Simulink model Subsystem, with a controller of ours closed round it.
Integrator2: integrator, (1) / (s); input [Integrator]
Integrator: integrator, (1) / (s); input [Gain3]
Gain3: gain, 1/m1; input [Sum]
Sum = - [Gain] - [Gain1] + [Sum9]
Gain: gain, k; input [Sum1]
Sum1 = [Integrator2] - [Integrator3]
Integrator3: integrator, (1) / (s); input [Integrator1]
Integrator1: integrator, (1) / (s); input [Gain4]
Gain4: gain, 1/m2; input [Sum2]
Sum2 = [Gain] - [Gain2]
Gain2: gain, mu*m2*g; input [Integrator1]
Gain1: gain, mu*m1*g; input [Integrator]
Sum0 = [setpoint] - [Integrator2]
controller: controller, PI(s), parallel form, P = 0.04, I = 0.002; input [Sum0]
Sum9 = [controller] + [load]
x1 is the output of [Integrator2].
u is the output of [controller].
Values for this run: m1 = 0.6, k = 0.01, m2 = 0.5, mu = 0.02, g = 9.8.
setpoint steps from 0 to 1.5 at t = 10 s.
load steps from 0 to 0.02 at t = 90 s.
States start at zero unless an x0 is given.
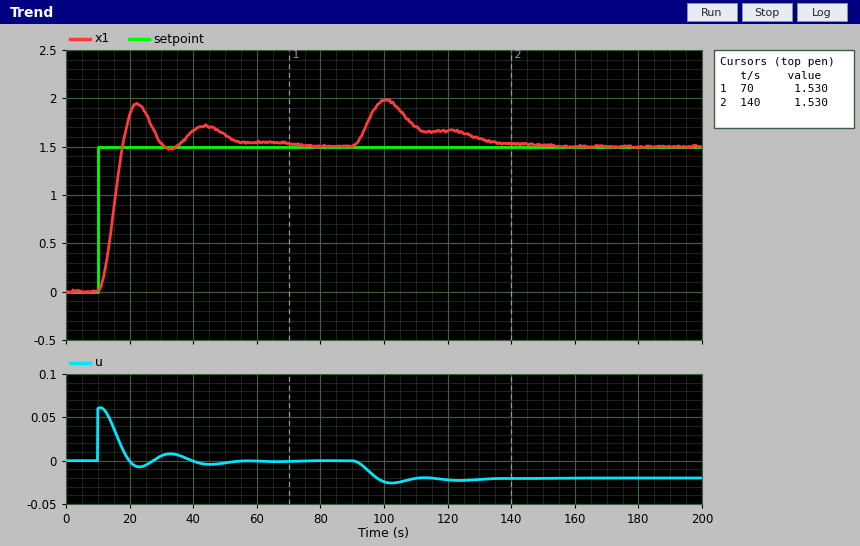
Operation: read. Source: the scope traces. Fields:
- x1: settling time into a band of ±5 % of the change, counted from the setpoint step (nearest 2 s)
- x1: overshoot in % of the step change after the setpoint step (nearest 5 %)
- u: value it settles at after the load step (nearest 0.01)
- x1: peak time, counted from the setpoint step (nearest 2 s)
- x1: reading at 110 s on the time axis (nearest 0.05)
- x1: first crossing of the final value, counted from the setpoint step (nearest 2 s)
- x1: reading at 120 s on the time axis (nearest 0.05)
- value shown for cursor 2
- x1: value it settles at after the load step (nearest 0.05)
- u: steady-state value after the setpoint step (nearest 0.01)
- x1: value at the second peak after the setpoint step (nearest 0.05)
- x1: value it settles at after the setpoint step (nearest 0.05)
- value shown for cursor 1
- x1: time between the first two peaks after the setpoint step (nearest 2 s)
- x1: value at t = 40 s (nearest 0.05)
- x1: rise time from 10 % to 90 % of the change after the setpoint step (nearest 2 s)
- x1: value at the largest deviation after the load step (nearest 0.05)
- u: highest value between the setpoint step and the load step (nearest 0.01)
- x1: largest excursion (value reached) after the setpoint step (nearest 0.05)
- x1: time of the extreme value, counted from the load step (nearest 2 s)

42 s
30 %
-0.02
12 s
1.70
8 s
1.65
1.530
1.50
0.00
1.70
1.50
1.530
22 s
1.65
6 s
2.00
0.06
1.95
10 s
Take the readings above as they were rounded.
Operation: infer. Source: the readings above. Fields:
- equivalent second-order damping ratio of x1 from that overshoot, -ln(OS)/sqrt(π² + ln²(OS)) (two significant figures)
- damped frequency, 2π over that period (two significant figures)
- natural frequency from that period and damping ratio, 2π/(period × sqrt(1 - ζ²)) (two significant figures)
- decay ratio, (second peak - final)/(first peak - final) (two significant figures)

0.36
0.29 rad/s
0.31 rad/s
0.44
